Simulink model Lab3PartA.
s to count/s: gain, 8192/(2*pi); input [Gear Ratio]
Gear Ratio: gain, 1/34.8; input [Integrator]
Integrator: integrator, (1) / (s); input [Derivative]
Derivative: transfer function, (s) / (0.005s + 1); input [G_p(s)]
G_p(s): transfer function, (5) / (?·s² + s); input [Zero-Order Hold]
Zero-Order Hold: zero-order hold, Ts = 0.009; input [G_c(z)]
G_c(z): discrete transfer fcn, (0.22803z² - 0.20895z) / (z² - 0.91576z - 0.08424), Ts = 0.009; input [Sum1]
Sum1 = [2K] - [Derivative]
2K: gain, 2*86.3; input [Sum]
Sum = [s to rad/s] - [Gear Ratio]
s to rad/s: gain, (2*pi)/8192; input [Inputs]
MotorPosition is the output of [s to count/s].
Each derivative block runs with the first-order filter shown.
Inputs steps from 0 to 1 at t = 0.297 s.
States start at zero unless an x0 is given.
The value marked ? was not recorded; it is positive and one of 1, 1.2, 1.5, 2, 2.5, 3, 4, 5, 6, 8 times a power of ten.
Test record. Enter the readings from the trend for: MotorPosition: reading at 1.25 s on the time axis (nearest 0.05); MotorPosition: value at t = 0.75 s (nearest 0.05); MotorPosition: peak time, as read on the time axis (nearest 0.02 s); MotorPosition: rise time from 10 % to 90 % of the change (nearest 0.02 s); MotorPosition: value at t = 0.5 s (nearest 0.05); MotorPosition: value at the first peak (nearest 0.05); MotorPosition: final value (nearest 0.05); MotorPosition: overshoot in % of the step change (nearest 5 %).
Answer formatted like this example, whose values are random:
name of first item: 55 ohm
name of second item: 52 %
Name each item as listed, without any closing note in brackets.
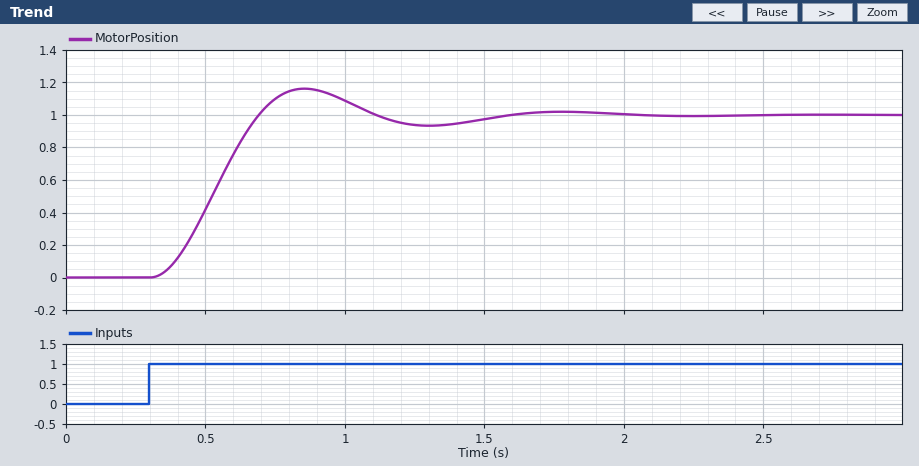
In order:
MotorPosition: reading at 1.25 s on the time axis: 0.95
MotorPosition: value at t = 0.75 s: 1.10
MotorPosition: peak time, as read on the time axis: 0.86 s
MotorPosition: rise time from 10 % to 90 % of the change: 0.26 s
MotorPosition: value at t = 0.5 s: 0.40
MotorPosition: value at the first peak: 1.15
MotorPosition: final value: 1.00
MotorPosition: overshoot in % of the step change: 15 %
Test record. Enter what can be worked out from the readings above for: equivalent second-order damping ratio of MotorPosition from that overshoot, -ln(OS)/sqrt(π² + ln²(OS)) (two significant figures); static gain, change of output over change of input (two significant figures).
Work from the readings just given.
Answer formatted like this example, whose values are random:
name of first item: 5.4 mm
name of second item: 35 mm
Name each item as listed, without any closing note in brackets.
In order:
equivalent second-order damping ratio of MotorPosition from that overshoot, -ln(OS)/sqrt(π² + ln²(OS)): 0.52
static gain, change of output over change of input: 1.0
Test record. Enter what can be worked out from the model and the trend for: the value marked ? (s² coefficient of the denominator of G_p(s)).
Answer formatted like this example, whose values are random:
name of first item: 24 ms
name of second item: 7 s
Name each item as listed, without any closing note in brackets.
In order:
the value marked ? (s² coefficient of the denominator of G_p(s)): 0.2
